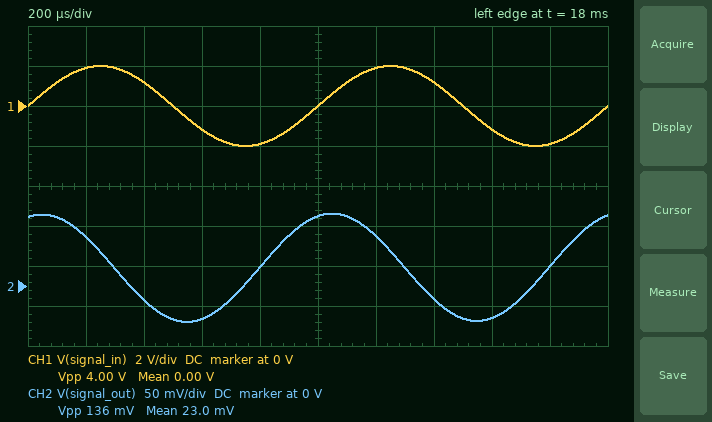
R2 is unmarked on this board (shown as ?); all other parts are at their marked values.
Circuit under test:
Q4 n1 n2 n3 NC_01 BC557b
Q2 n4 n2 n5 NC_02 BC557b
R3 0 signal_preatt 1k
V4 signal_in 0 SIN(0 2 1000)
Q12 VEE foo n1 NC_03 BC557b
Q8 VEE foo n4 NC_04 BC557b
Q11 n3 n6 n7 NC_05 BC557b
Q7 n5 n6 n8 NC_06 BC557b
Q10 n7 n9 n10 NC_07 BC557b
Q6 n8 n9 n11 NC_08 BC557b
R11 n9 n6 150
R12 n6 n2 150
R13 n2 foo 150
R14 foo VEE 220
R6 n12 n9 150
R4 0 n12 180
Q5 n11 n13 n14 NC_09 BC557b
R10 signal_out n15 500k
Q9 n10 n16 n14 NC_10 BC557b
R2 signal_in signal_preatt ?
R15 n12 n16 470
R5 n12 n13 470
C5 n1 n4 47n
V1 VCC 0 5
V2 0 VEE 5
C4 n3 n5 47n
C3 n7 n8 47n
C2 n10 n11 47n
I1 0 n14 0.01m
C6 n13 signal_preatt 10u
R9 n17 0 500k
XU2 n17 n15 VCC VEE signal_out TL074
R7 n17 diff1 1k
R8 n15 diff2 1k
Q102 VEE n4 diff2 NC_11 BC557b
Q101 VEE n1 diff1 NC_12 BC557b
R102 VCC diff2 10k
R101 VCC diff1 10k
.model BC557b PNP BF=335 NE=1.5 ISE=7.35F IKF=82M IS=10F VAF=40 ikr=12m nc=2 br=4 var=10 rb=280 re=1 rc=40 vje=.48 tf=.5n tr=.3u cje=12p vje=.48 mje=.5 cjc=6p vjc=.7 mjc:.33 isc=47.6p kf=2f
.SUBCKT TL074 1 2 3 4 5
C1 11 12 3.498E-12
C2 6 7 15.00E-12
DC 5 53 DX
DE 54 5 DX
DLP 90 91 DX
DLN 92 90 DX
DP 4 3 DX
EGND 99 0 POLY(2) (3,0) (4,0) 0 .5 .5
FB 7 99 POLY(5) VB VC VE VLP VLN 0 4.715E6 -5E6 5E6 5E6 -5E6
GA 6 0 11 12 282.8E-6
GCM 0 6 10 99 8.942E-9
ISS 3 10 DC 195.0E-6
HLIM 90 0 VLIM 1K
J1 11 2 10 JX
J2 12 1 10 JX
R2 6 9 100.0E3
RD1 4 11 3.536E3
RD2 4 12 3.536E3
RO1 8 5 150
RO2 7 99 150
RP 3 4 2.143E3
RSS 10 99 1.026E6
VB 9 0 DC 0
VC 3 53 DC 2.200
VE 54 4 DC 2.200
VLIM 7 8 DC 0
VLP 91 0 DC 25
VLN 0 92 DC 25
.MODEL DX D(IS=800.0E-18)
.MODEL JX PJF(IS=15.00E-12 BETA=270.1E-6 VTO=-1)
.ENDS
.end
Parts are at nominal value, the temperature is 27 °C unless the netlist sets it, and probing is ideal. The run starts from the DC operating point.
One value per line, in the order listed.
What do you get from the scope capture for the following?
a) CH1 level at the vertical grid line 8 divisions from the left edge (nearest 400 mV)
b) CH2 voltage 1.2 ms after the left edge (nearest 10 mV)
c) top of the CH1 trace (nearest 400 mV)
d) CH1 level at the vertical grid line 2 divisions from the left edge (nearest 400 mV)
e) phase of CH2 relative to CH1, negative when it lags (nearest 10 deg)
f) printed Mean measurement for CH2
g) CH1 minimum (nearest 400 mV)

-1.2 V
60 mV
2.0 V
1.2 V
70 deg
23.0 mV
-2.0 V
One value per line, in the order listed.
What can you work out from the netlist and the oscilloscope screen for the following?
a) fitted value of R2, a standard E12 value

33 kΩ
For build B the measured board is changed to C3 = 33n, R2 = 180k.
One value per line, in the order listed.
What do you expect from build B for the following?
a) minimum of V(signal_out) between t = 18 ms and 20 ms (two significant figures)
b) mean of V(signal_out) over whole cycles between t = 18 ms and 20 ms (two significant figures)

20 mV
37 mV
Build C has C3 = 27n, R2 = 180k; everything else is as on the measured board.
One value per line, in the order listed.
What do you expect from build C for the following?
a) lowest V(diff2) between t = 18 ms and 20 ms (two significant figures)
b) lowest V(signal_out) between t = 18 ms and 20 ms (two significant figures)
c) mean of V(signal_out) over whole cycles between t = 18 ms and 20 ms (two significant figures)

-2.7 V
17 mV
37 mV
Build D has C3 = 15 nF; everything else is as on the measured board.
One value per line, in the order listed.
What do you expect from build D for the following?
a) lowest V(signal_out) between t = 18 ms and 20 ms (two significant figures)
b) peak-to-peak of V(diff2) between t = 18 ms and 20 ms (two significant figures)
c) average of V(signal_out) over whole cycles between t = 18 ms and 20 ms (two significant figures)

-130 mV
3.0 mV
23 mV
